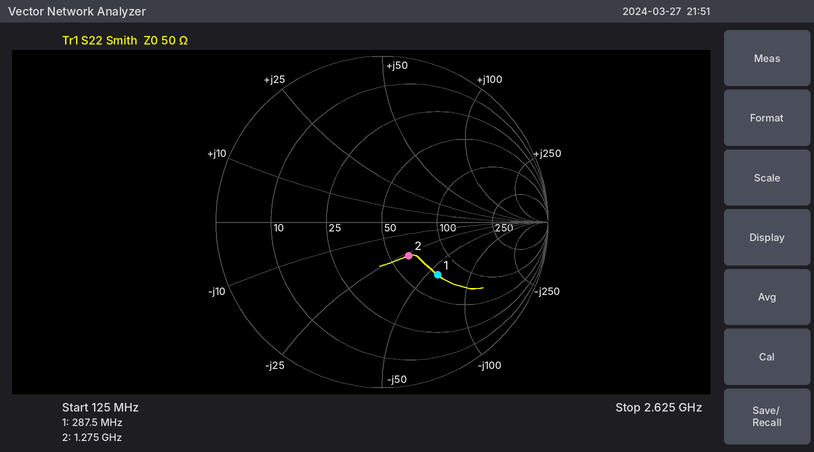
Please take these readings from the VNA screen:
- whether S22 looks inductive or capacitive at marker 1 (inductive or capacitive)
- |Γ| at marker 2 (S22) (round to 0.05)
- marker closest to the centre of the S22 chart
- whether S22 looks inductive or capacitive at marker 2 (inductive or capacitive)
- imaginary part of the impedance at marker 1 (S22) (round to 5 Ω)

capacitive
0.25
marker 2
capacitive
-60 Ω
